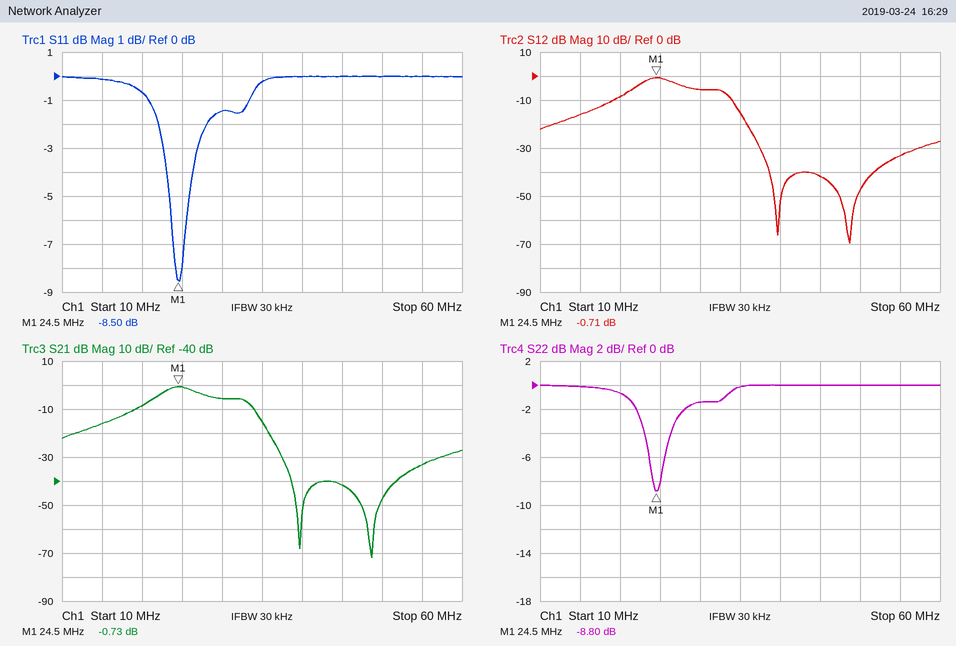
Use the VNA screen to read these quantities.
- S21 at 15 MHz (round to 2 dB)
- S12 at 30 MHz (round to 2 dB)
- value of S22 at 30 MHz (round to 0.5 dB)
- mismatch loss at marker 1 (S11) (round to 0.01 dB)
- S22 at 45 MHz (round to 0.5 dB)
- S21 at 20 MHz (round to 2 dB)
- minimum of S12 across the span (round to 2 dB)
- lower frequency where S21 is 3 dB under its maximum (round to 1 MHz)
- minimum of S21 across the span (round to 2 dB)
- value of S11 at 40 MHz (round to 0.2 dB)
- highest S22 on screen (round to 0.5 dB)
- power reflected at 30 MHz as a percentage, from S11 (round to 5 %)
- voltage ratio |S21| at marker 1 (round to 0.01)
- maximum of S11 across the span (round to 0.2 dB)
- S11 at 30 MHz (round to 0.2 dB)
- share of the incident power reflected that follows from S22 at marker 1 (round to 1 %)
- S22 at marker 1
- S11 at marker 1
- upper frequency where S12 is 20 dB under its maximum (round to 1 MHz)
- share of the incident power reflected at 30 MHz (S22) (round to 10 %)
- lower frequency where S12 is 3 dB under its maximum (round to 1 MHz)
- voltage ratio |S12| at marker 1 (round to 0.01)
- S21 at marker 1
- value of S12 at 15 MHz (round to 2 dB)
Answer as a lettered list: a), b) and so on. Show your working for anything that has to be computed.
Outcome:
a) -16 dB
b) -6 dB
c) -1.5 dB
d) −10 log10(1 − 10^(-8.5/10)) ≈ 0.66 dB
e) 0.0 dB
f) -8 dB
g) -70 dB
h) 22 MHz
i) -72 dB
j) 0.0 dB
k) 0.0 dB
l) 10^(-1.4/10) ≈ 72.4 %, so 70 % to the nearest 5 %
m) 10^(-0.73/20) ≈ 0.92
n) 0.0 dB
o) -1.4 dB
p) 10^(-8.8/10) ≈ 13 %
q) -8.80 dB
r) -8.50 dB
s) 36 MHz
t) 10^(-1.5/10) ≈ 70.8 %, so 70 % to the nearest 10 %
u) 22 MHz
v) 10^(-0.71/20) ≈ 0.92
w) -0.73 dB
x) -16 dB
